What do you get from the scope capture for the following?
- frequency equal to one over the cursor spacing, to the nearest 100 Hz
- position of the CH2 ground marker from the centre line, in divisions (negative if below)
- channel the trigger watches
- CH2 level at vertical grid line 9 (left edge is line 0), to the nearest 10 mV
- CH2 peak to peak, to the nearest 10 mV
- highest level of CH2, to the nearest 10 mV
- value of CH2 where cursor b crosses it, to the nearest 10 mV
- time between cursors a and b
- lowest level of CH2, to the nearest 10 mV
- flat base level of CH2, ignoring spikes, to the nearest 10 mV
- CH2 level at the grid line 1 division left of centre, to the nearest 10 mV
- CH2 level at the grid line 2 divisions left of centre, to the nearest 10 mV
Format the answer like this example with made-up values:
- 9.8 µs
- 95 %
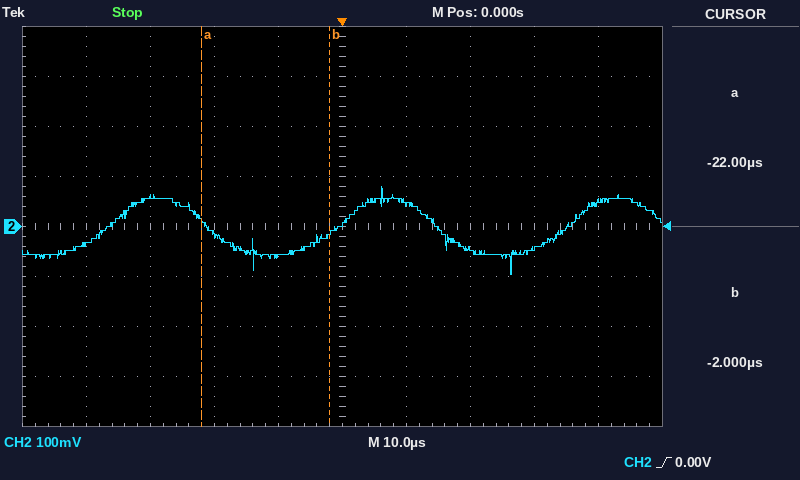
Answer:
- 50.0 kHz
- 0.0 div
- CH2
- 50 mV
- 180 mV
- 80 mV
- -20 mV
- 20 µs
- -100 mV
- -60 mV
- -60 mV
- -20 mV
